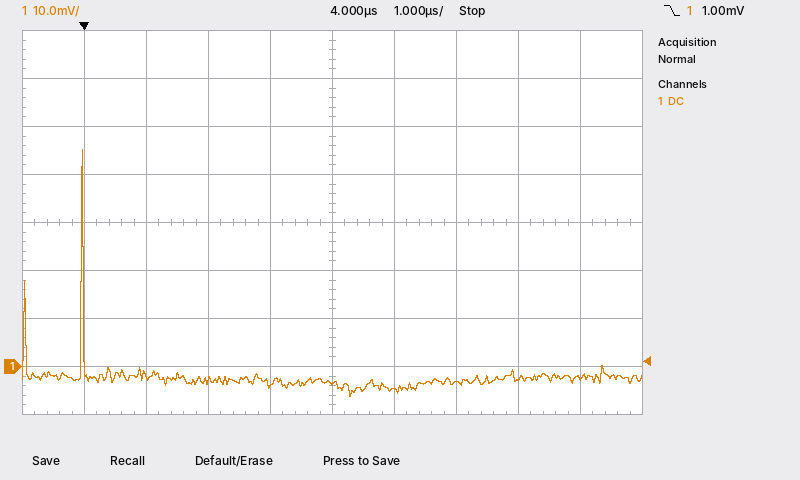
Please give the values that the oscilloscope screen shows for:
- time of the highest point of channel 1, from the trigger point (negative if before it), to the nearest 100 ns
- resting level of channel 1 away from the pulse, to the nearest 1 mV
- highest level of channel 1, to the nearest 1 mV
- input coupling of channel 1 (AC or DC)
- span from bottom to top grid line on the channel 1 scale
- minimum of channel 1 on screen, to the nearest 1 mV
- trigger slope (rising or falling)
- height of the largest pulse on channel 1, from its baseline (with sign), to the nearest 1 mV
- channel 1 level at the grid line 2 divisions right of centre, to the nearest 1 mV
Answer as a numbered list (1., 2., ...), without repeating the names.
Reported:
1. 0.0 µs
2. -3 mV
3. 45 mV
4. DC
5. 80 mV
6. -6 mV
7. falling
8. +48 mV
9. -3 mV
